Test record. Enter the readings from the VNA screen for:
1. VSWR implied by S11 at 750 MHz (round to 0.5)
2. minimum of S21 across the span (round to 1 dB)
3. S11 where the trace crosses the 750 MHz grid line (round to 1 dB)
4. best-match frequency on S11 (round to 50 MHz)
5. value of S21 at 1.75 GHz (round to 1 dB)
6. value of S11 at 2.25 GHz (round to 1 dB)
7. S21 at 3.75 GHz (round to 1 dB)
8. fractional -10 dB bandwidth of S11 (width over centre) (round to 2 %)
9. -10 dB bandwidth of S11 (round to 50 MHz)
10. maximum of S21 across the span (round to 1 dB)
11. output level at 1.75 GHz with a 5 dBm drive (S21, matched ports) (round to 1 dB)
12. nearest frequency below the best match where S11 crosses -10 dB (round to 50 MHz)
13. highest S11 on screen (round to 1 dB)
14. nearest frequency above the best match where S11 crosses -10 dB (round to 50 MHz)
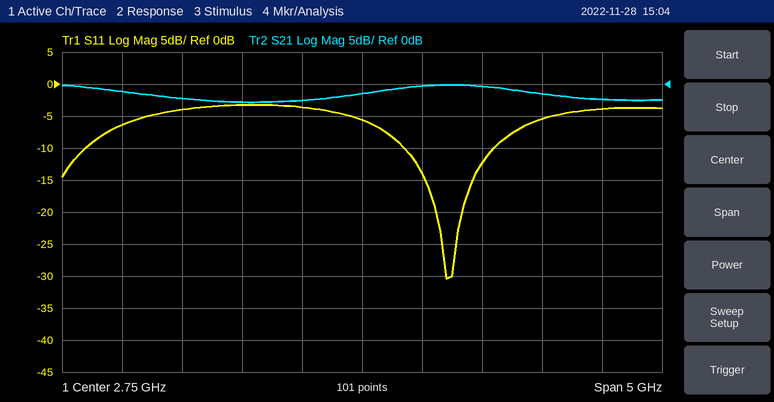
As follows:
3.0
-3 dB
-6 dB
3.45 GHz
-3 dB
-4 dB
0 dB
22 %
750 MHz
0 dB
2 dBm
3.10 GHz
-3 dB
3.85 GHz
